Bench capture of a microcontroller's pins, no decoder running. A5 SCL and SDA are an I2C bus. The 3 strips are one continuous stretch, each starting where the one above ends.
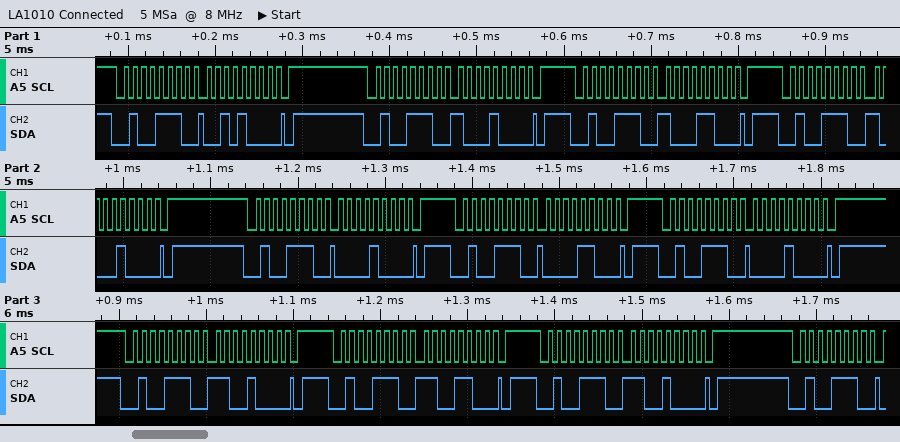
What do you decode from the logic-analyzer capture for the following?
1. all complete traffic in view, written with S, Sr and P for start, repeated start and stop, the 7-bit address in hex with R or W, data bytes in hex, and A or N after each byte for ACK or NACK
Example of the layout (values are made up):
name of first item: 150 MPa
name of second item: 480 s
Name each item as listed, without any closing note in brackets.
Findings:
all complete traffic in view, written with S, Sr and P for start, repeated start and stop, the 7-bit address in hex with R or W, data bytes in hex, and A or N after each byte for ACK or NACK: S 27W A 28 A P S 27W A 88 A P S 27W A 8C A P S 27W A 88 A P S 27W A 08 A P S 27W A 0C A P S 27W A 08 A P S 27W A C8 A P S 27W A CC A P S 27W A C8 A P S 27W A
